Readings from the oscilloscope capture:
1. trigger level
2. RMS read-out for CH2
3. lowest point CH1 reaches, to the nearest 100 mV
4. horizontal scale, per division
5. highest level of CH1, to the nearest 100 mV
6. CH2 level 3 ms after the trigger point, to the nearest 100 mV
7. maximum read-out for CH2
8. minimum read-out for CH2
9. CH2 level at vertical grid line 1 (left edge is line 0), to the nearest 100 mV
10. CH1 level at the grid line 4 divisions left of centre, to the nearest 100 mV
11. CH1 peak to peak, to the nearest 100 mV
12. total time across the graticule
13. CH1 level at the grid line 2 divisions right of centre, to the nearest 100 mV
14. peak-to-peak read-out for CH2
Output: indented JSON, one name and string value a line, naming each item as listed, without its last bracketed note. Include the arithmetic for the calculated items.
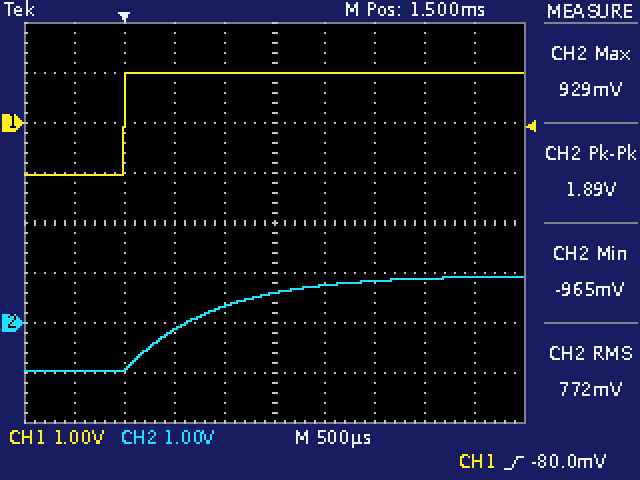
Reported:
{
  "trigger level": "-80.0 mV",
  "RMS read-out for CH2": "772 mV",
  "lowest point CH1 reaches, to the nearest 100 mV": "-1.0 V",
  "horizontal scale, per division": "500 µs",
  "highest level of CH1, to the nearest 100 mV": "1.0 V",
  "CH2 level 3 ms after the trigger point, to the nearest 100 mV": "900 mV",
  "maximum read-out for CH2": "929 mV",
  "minimum read-out for CH2": "-965 mV",
  "CH2 level at vertical grid line 1 (left edge is line 0), to the nearest 100 mV": "-1.0 V",
  "CH1 level at the grid line 4 divisions left of centre, to the nearest 100 mV": "-1.0 V",
  "CH1 peak to peak, to the nearest 100 mV": "1.0 V − (-1.0 V) = 2.0 V",
  "total time across the graticule": "5 ms",
  "CH1 level at the grid line 2 divisions right of centre, to the nearest 100 mV": "1.0 V",
  "peak-to-peak read-out for CH2": "1.89 V"
}
